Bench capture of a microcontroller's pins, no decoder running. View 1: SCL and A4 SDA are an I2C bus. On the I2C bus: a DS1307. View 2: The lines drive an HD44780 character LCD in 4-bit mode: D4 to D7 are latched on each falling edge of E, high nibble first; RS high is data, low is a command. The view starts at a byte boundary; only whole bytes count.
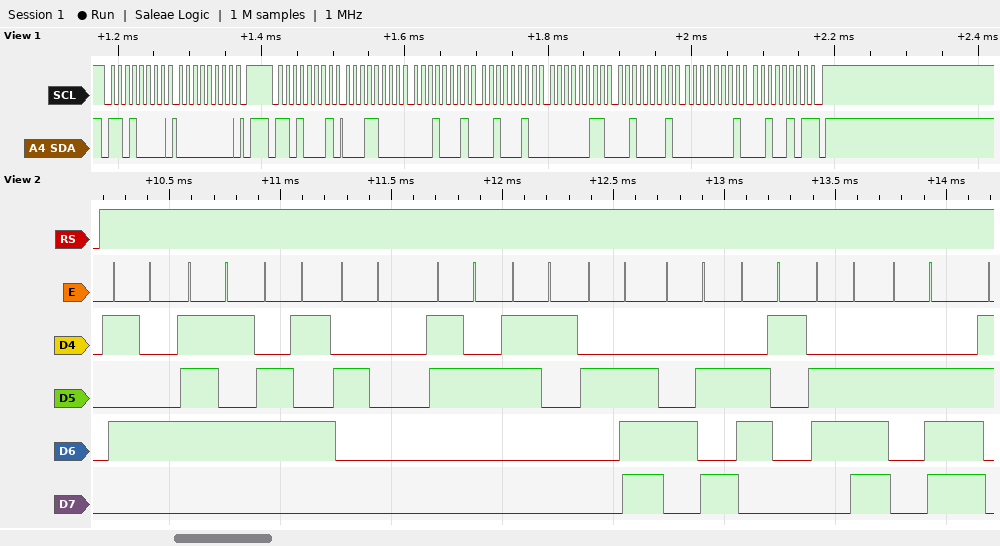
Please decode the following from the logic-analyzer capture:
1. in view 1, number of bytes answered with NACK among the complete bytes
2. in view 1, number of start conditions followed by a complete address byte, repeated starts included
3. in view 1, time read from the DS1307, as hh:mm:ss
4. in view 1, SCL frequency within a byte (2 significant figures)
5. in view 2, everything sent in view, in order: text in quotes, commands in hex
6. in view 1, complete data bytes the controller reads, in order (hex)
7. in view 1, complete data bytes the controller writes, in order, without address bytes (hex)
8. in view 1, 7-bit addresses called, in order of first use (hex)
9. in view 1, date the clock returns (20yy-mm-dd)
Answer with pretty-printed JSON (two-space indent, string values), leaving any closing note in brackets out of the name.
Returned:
{
  "in view 1, number of bytes answered with NACK among the complete bytes": "1",
  "in view 1, number of start conditions followed by a complete address byte, repeated starts included": "2",
  "in view 1, time read from the DS1307, as hh:mm:ss": "22:11:18",
  "in view 1, SCL frequency within a byte": "100 kHz",
  "in view 2, everything sent in view, in order: text in quotes, commands in hex": "\"Tue 21.Jan.\"",
  "in view 1, complete data bytes the controller reads, in order": "18 11 22 03 21 01 25",
  "in view 1, complete data bytes the controller writes, in order, without address bytes": "00",
  "in view 1, 7-bit addresses called, in order of first use": "0x68",
  "in view 1, date the clock returns": "2025-01-21"
}
